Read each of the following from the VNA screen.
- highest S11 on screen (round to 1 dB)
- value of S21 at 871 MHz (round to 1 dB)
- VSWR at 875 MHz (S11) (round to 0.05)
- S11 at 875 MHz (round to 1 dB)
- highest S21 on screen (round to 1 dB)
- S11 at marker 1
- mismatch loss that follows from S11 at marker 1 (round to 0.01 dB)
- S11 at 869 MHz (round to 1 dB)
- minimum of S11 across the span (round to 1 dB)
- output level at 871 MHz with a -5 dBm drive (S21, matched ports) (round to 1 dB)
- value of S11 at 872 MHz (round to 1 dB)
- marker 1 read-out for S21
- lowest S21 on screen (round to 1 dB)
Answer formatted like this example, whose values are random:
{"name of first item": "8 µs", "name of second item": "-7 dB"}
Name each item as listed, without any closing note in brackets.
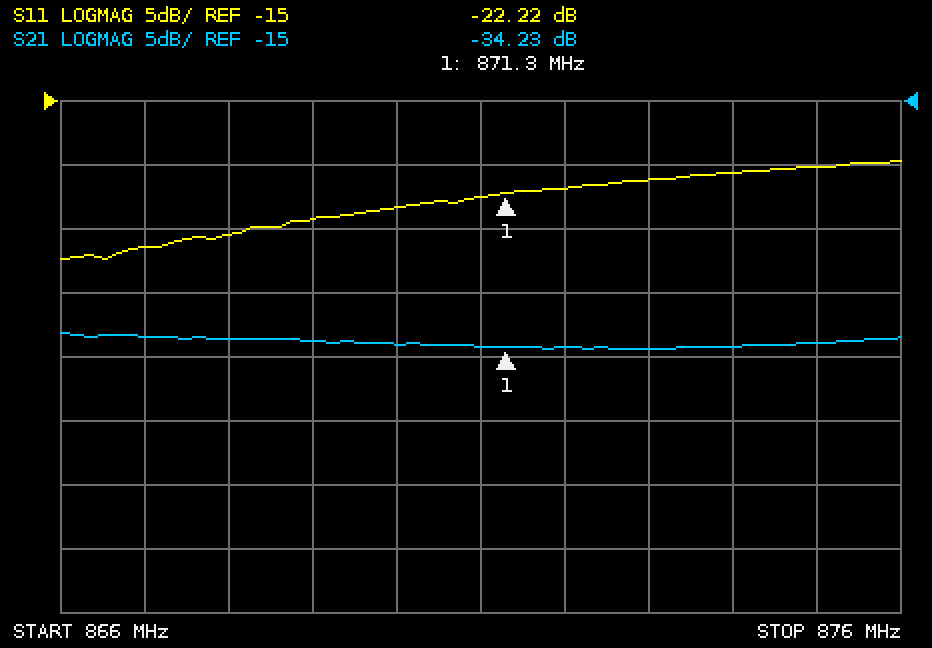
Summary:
{"highest S11 on screen": "-20 dB", "value of S21 at 871 MHz": "-34 dB", "VSWR at 875 MHz (S11)": "1.20", "S11 at 875 MHz": "-20 dB", "highest S21 on screen": "-33 dB", "S11 at marker 1": "-22.22 dB", "mismatch loss that follows from S11 at marker 1": "0.03 dB", "S11 at 869 MHz": "-24 dB", "minimum of S11 across the span": "-27 dB", "output level at 871 MHz with a -5 dBm drive (S21, matched ports)": "-39 dBm", "value of S11 at 872 MHz": "-22 dB", "marker 1 read-out for S21": "-34.23 dB", "lowest S21 on screen": "-34 dB"}
